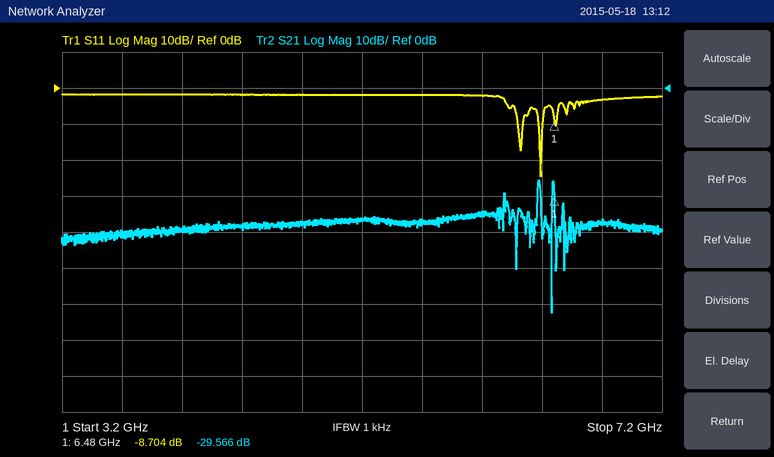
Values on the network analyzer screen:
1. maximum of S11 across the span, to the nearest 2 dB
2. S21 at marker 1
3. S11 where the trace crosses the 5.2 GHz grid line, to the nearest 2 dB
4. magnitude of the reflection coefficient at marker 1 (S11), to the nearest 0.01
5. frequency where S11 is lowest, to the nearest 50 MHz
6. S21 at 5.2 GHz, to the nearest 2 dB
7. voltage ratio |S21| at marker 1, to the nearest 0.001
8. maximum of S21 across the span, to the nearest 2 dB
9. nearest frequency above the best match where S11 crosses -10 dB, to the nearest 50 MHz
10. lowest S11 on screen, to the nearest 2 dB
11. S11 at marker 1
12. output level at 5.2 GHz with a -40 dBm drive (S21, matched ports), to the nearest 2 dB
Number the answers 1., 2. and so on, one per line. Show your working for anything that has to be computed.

1. -2 dB
2. -29.566 dB
3. -2 dB
4. 10^(-8.704/20) ≈ 0.37
5. 6.40 GHz
6. -36 dB
7. 10^(-29.566/20) ≈ 0.033
8. -26 dB
9. 6.40 GHz
10. -24 dB
11. -8.704 dB
12. -40 dBm + (-36 dB) = -76 dBm
